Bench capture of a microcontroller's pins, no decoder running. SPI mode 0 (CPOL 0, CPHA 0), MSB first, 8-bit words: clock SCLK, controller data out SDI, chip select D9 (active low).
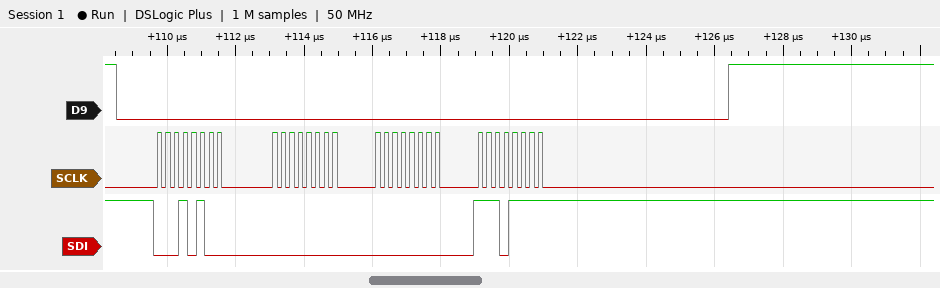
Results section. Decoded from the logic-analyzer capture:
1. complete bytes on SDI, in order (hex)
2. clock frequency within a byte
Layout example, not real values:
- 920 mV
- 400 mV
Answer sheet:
- 14 00 00 EF
- 4 MHz
